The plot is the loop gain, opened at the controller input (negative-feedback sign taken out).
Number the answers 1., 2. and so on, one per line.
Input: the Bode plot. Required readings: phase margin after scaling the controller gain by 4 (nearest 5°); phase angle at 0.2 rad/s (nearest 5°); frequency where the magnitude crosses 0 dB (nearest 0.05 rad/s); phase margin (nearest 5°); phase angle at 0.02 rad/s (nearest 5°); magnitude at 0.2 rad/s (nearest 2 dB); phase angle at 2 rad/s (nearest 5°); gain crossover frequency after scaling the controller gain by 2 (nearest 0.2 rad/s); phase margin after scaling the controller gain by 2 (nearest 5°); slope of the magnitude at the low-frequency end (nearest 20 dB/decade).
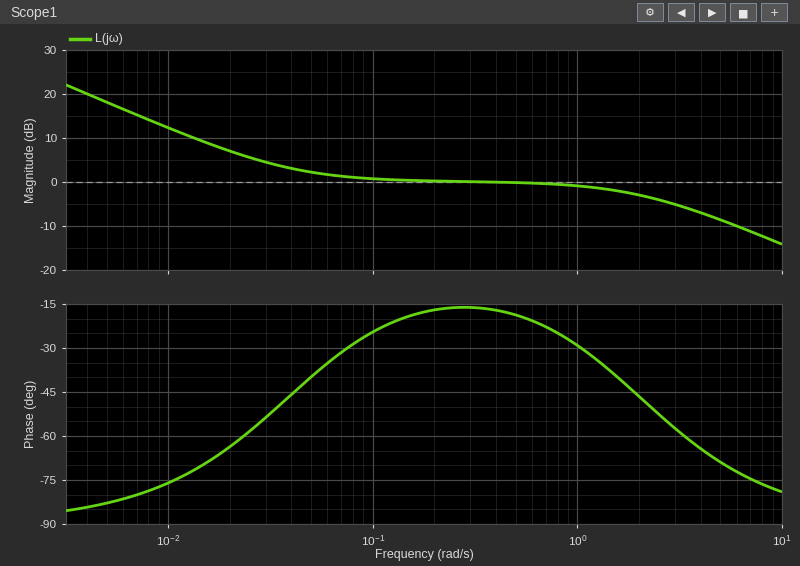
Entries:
1. 105°
2. -15°
3. 0.40 rad/s
4. 165°
5. -65°
6. 0 dB
7. -45°
8. 3.4 rad/s
9. 120°
10. -20 dB/decade
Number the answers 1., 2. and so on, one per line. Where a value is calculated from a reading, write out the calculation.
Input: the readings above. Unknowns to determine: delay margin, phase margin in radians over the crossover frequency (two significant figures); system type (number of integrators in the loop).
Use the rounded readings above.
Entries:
1. 165 × π / 180 / 0.4 = 7.2 s
2. 1
